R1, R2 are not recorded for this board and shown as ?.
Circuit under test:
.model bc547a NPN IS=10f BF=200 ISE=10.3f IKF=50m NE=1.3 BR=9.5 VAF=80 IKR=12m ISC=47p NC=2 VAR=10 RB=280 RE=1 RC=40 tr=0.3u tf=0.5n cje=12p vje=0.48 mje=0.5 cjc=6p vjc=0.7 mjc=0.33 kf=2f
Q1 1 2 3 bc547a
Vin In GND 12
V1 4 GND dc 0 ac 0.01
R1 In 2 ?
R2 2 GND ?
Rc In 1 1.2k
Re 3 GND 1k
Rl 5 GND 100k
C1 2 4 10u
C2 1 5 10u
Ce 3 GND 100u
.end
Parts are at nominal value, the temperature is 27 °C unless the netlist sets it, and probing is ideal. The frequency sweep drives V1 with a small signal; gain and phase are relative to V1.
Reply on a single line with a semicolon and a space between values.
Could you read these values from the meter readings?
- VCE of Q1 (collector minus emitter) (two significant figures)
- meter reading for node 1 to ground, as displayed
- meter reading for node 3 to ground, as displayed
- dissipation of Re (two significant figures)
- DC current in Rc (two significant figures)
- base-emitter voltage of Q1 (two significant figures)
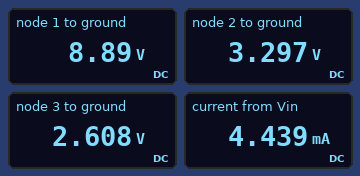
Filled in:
6.3 V; 8.89 V; 2.608 V; 6.8 mW; 2.6 mA; 690 mV
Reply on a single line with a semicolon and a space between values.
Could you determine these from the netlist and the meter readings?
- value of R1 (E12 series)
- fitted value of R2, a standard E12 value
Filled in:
4.7 kΩ; 1.8 kΩ
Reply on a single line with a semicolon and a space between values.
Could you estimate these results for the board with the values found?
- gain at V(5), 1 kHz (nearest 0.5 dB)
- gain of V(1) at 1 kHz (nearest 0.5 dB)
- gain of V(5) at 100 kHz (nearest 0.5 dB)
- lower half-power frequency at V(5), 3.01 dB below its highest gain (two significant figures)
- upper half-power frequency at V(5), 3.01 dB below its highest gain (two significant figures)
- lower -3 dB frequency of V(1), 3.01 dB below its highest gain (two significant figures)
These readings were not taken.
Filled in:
38.5 dB; 38.5 dB; 38.5 dB; 130 Hz; 1.7 MHz; 130 Hz
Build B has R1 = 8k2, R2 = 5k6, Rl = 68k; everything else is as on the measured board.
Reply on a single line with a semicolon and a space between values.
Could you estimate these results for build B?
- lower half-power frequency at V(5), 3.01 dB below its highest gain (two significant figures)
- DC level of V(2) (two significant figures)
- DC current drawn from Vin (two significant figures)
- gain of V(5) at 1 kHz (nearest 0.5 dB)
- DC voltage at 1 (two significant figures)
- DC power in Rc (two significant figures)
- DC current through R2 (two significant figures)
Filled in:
160 Hz; 4.8 V; 4.9 mA; 40.5 dB; 7.2 V; 19 mW; 850 µA
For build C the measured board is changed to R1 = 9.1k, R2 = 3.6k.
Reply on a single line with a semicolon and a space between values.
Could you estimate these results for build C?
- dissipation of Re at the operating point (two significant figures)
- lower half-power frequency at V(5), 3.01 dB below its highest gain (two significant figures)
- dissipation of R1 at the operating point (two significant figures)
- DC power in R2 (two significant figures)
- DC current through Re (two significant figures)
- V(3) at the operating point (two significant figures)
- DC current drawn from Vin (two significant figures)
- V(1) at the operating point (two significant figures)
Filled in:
7.1 mW; 130 Hz; 8.2 mW; 3.1 mW; 2.7 mA; 2.7 V; 3.6 mA; 8.8 V
